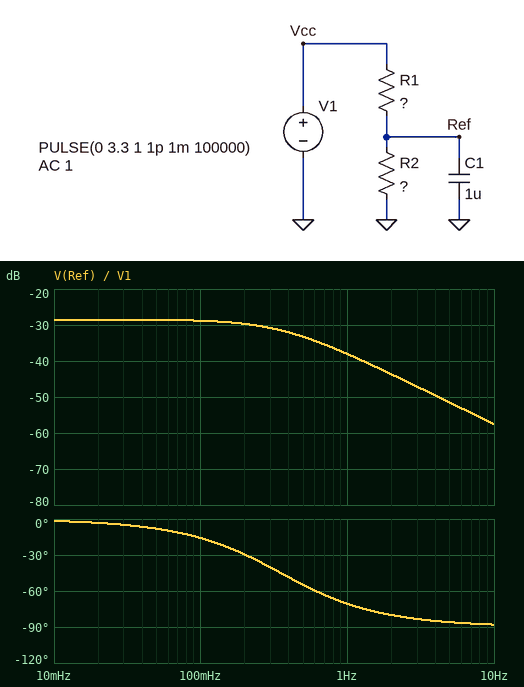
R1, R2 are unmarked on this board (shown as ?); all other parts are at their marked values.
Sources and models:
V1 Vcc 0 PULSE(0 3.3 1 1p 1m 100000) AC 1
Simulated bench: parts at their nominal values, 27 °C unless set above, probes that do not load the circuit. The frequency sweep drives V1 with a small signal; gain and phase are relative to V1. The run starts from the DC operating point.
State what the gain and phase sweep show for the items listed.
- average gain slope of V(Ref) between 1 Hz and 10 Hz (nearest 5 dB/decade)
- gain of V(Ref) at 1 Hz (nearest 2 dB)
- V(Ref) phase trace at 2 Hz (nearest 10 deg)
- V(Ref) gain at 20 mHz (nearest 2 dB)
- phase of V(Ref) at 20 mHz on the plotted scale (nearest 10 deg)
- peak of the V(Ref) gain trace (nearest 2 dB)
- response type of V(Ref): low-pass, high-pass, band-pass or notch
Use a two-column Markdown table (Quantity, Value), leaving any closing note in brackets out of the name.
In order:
| Quantity | Value |
|---|---|
| average gain slope of V(Ref) between 1 Hz and 10 Hz | -20 dB/decade |
| gain of V(Ref) at 1 Hz | -38 dB |
| V(Ref) phase trace at 2 Hz | -80 deg |
| V(Ref) gain at 20 mHz | -28 dB |
| phase of V(Ref) at 20 mHz on the plotted scale | 0 deg |
| peak of the V(Ref) gain trace | -28 dB |
| response type of V(Ref): low-pass, high-pass, band-pass or notch | low-pass |
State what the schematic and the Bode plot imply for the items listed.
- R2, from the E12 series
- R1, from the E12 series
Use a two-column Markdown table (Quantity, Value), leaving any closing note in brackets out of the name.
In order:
| Quantity | Value |
|---|---|
| R2, from the E12 series | 470 kΩ |
| R1, from the E12 series | 12 MΩ |
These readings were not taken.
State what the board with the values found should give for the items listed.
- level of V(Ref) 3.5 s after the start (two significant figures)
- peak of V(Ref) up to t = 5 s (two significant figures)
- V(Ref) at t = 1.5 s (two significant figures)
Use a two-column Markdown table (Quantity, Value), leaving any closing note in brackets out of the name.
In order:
| Quantity | Value |
|---|---|
| level of V(Ref) 3.5 s after the start | 120 mV |
| peak of V(Ref) up to t = 5 s | 120 mV |
| V(Ref) at t = 1.5 s | 83 mV |
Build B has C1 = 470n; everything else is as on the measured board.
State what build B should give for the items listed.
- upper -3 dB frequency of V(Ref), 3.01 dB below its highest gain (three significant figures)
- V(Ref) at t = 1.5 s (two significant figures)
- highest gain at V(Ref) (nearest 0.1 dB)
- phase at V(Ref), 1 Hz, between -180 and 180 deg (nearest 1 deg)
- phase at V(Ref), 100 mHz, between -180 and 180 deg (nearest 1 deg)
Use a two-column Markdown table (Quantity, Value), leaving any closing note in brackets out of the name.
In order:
| Quantity | Value |
|---|---|
| upper -3 dB frequency of V(Ref), 3.01 dB below its highest gain | 749 mHz |
| V(Ref) at t = 1.5 s | 110 mV |
| highest gain at V(Ref) | -28.5 dB |
| phase at V(Ref), 1 Hz, between -180 and 180 deg | -53 deg |
| phase at V(Ref), 100 mHz, between -180 and 180 deg | -8 deg |
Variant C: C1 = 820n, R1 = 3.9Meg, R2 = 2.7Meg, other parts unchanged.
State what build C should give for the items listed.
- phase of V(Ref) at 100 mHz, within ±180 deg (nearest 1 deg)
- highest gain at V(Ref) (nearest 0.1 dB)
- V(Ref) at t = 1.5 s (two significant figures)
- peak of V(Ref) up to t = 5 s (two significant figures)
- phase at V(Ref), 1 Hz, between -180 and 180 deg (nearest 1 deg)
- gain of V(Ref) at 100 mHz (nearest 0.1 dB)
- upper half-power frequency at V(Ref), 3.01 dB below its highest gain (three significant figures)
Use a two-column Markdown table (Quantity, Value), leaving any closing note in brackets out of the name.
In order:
| Quantity | Value |
|---|---|
| phase of V(Ref) at 100 mHz, within ±180 deg | -39 deg |
| highest gain at V(Ref) | -7.8 dB |
| V(Ref) at t = 1.5 s | 430 mV |
| peak of V(Ref) up to t = 5 s | 1.3 V |
| phase at V(Ref), 1 Hz, between -180 and 180 deg | -83 deg |
| gain of V(Ref) at 100 mHz | -10.0 dB |
| upper half-power frequency at V(Ref), 3.01 dB below its highest gain | 122 mHz |
